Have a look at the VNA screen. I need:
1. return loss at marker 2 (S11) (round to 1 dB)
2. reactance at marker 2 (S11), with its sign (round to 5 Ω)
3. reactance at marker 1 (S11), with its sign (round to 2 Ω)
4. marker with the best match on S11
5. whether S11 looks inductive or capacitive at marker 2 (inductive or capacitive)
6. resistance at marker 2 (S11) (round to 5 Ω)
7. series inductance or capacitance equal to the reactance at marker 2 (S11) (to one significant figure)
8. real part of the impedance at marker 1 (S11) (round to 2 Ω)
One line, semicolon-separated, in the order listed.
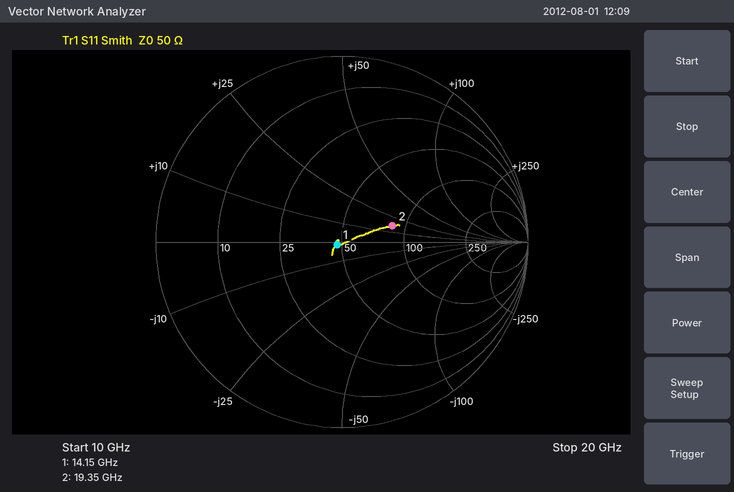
11 dB; +15 Ω; -2 Ω; marker 1; inductive; 85 Ω; 100 pH; 48 Ω
